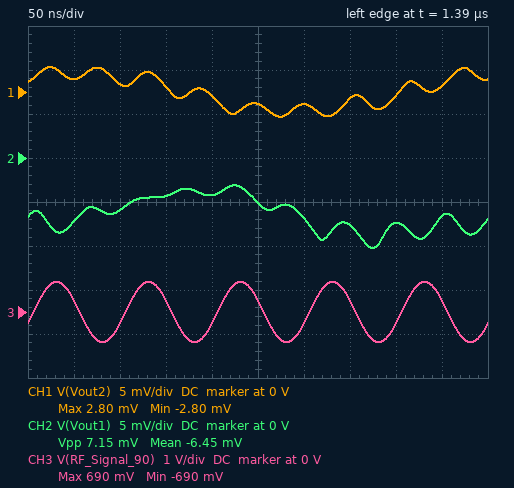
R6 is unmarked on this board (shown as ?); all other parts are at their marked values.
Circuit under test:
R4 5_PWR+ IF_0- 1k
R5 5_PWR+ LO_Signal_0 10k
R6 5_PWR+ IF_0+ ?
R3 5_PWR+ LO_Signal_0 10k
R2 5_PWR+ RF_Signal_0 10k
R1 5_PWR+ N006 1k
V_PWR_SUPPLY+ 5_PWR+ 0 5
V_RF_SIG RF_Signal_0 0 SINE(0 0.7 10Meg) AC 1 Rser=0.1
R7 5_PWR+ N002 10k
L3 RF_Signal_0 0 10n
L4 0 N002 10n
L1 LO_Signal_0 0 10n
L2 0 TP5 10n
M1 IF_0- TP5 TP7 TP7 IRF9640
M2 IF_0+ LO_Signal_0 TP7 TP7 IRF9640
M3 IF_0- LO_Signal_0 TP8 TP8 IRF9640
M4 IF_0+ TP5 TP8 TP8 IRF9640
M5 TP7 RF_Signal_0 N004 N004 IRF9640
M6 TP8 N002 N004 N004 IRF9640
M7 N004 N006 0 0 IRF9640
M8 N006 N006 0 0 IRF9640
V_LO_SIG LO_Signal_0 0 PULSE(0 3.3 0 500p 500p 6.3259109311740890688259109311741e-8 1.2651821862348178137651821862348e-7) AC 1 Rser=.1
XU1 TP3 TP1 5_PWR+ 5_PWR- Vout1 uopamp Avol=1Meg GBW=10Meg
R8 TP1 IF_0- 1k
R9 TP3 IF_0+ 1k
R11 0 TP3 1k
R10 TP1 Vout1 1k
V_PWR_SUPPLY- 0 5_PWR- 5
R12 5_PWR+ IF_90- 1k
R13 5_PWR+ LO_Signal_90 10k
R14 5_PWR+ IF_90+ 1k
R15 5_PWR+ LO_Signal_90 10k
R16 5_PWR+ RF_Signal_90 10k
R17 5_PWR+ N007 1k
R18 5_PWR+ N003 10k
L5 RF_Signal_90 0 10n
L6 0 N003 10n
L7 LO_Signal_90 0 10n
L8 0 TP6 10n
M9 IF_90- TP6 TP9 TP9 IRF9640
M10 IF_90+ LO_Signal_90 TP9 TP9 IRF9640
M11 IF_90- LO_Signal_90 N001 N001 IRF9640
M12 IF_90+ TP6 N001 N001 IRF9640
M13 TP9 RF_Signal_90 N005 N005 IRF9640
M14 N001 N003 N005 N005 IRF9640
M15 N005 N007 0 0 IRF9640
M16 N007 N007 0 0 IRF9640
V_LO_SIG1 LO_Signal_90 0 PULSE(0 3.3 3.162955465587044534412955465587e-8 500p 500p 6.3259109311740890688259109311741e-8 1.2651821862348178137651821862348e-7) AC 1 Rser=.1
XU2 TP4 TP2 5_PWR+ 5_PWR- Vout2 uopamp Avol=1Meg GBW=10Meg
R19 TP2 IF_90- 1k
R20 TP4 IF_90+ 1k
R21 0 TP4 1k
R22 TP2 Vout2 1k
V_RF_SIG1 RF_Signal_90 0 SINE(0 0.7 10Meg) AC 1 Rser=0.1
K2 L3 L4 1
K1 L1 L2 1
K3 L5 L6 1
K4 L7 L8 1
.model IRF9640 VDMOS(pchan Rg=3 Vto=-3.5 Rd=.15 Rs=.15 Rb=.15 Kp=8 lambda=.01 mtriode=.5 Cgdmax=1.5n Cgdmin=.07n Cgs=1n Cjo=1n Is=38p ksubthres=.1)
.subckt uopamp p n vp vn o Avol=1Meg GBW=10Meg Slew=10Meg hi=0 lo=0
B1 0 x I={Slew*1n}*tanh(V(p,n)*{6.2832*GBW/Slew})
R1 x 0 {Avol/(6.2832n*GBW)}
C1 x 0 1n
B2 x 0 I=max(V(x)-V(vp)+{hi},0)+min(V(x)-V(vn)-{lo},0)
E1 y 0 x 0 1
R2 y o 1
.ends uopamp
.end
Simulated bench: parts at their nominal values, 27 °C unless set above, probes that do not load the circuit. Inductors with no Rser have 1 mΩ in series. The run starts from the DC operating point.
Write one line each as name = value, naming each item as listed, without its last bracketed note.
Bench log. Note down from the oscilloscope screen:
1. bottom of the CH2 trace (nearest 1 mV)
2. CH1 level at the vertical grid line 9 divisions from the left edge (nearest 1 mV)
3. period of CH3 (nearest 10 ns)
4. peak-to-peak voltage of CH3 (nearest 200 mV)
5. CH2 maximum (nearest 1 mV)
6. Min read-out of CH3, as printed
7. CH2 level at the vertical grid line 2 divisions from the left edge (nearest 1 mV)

bottom of the CH2 trace = -10 mV
CH1 level at the vertical grid line 9 divisions from the left edge = 1 mV
period of CH3 = 100 ns
peak-to-peak voltage of CH3 = 1.4 V
CH2 maximum = -3 mV
Min read-out of CH3, as printed = -690 mV
CH2 level at the vertical grid line 2 divisions from the left edge = -6 mV
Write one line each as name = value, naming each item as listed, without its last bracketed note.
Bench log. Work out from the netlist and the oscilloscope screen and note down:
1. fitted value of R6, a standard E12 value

fitted value of R6, a standard E12 value = 1.2 kΩ
